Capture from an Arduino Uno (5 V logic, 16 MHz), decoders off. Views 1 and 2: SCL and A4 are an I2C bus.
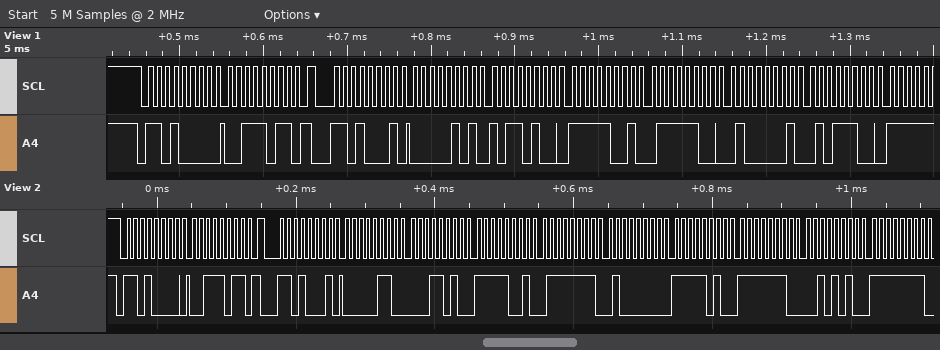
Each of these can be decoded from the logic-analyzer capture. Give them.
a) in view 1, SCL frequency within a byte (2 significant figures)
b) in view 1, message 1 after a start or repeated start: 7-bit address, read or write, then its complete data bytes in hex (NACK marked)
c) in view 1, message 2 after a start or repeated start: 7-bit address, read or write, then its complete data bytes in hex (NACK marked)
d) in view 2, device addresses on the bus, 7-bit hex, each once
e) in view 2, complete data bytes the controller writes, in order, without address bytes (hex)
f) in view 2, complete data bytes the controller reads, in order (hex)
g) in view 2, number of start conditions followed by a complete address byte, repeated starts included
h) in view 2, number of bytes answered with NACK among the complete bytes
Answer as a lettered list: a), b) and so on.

a) 100 kHz
b) 0x68 write: 3B
c) 0x68 read: 05 B4 F9 7C 41 5C
d) 0x68
e) 3B
f) 06 1A F9 7F 40 FA FE 2A FF
g) 2
h) 0
